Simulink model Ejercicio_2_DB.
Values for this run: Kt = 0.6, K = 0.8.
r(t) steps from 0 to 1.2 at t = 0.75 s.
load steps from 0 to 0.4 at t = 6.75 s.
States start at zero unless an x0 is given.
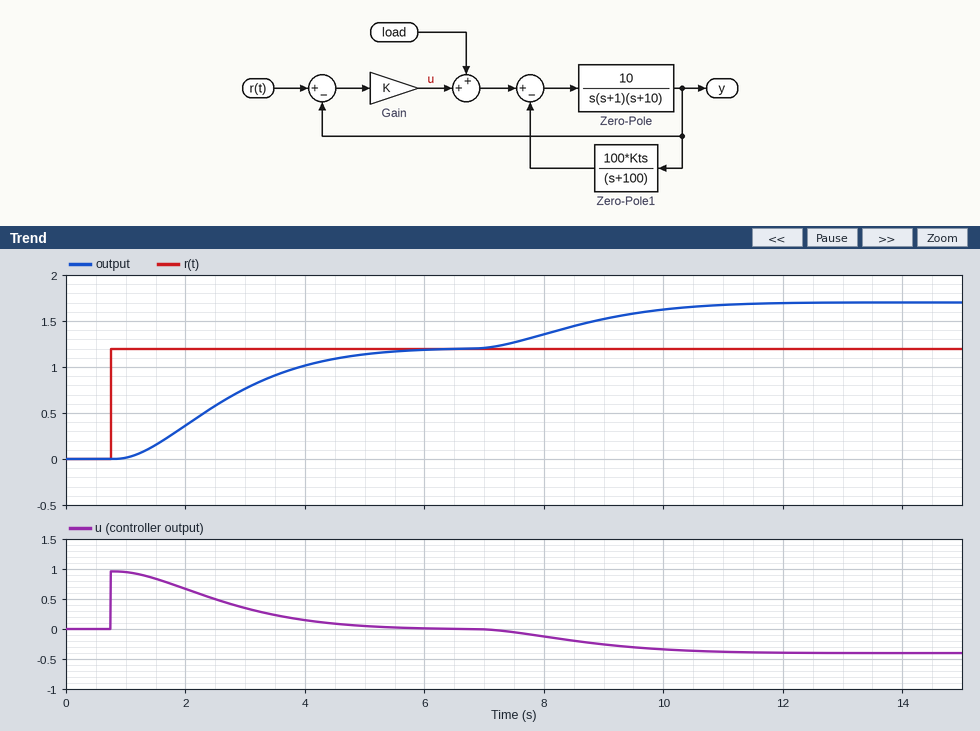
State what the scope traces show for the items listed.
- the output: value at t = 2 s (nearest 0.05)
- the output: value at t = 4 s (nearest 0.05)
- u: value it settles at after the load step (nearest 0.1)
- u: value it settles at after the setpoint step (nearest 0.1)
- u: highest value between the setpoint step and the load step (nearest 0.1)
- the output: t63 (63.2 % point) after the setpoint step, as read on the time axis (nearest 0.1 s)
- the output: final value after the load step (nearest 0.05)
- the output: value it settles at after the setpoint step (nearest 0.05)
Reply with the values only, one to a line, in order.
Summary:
0.35
1.00
-0.4
0.0
1.0
3.0 s
1.70
1.20
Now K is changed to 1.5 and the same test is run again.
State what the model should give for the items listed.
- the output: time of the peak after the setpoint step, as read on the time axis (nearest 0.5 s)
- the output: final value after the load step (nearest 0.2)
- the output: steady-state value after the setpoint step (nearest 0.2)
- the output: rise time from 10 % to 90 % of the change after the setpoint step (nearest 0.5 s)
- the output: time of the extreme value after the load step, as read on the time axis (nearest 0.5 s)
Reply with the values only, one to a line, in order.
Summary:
4.0 s
1.4
1.2
1.5 s
10.0 s
